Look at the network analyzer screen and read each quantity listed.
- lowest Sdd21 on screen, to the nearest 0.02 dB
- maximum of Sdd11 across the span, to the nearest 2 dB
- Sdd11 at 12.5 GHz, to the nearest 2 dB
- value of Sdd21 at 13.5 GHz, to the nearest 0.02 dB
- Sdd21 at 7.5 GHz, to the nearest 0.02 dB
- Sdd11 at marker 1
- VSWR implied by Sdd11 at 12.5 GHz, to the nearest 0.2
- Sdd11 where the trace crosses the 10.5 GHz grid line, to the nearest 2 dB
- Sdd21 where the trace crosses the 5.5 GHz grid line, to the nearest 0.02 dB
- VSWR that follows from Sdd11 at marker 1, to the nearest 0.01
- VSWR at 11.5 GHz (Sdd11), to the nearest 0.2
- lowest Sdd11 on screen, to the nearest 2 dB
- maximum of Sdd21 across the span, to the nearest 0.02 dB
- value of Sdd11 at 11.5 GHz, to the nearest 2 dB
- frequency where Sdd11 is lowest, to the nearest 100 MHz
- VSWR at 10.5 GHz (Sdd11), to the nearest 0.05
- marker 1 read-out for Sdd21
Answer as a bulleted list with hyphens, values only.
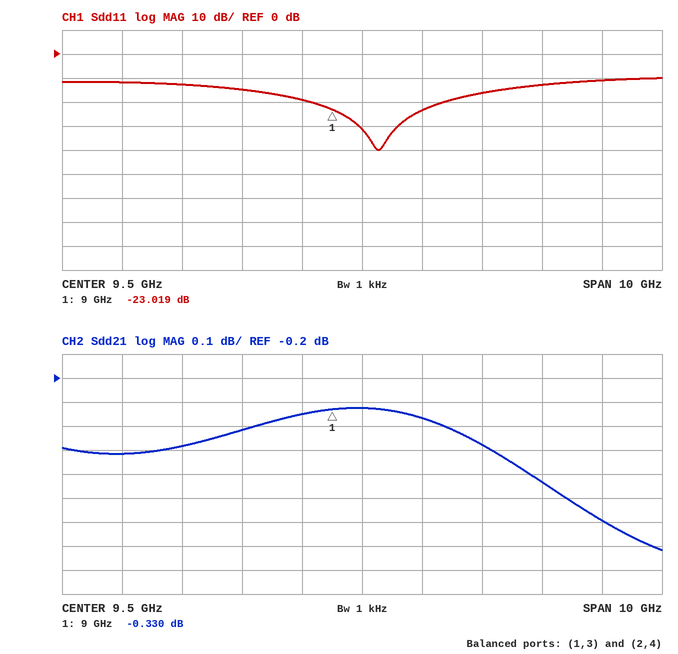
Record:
- -0.92 dB
- -10 dB
- -12 dB
- -0.80 dB
- -0.42 dB
- -23.019 dB
- 1.6
- -24 dB
- -0.52 dB
- 1.15
- 1.4
- -40 dB
- -0.32 dB
- -16 dB
- 9.8 GHz
- 1.15
- -0.330 dB
